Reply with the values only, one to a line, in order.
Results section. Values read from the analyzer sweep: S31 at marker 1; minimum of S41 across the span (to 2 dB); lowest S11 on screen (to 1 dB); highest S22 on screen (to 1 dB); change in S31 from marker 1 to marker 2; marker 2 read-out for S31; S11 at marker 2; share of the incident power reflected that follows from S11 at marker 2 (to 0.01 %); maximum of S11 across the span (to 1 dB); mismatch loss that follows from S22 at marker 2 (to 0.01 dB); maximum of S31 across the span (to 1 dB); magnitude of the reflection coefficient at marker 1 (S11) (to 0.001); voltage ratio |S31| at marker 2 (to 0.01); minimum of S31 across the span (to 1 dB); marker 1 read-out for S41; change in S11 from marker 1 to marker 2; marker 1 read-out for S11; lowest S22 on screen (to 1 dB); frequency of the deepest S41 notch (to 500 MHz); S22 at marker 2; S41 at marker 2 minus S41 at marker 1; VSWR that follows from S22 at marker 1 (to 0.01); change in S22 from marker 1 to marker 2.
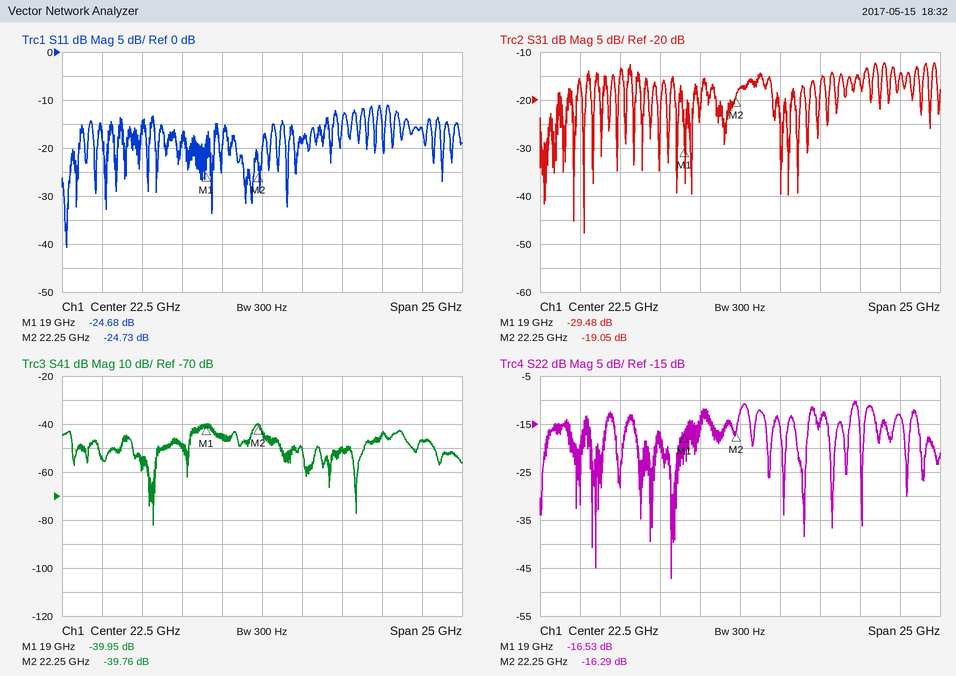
-29.48 dB
-82 dB
-41 dB
-10 dB
10.43 dB
-19.05 dB
-24.73 dB
0.34 %
-11 dB
0.10 dB
-12 dB
0.058
0.11
-48 dB
-39.95 dB
-0.05 dB
-24.68 dB
-47 dB
15.5 GHz
-16.29 dB
0.19 dB
1.35
0.24 dB
